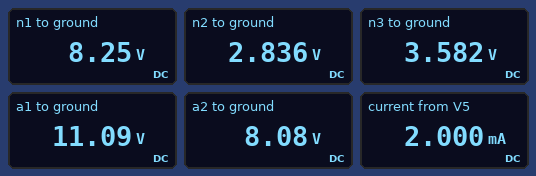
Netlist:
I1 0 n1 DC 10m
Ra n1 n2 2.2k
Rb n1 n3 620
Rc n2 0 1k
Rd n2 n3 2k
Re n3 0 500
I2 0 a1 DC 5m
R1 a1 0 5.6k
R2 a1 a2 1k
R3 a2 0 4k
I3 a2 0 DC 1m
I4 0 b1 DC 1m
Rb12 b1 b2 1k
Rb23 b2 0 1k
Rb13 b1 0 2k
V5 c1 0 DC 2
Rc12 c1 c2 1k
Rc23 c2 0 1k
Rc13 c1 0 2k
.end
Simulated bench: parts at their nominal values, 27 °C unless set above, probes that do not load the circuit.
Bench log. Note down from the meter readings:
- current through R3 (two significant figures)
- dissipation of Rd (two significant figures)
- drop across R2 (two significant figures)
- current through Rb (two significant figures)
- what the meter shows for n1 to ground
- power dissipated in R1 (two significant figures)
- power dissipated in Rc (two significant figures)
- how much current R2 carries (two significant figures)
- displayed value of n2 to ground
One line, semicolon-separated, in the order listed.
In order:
2.0 mA; 280 µW; 3.0 V; 7.5 mA; 8.25 V; 22 mW; 8.0 mW; 3.0 mA; 2.836 V
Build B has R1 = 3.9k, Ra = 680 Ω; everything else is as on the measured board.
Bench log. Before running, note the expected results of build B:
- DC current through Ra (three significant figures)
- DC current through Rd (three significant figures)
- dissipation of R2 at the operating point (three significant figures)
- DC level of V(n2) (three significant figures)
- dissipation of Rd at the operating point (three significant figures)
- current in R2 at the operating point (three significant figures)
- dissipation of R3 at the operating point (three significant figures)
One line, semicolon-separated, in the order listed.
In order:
4.20 mA; 371 µA; 6.97 mW; 3.83 V; 275 µW; 2.64 mA; 10.8 mW
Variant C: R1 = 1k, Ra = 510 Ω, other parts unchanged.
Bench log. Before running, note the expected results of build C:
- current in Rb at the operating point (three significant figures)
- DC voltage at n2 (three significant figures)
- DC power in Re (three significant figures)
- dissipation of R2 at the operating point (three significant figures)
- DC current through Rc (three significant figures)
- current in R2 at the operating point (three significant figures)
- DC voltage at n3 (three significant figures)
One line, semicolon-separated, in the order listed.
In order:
5.44 mA; 4.03 V; 17.8 mW; 2.25 mW; 4.03 mA; 1.50 mA; 2.98 V
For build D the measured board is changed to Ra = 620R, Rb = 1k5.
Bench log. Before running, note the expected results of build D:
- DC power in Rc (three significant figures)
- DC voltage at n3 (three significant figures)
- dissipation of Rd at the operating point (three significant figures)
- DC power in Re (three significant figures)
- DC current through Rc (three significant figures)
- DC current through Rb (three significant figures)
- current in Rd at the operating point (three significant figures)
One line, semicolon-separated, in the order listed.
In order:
23.6 mW; 2.57 V; 2.61 mW; 13.2 mW; 4.86 mA; 4.00 mA; 1.14 mA
